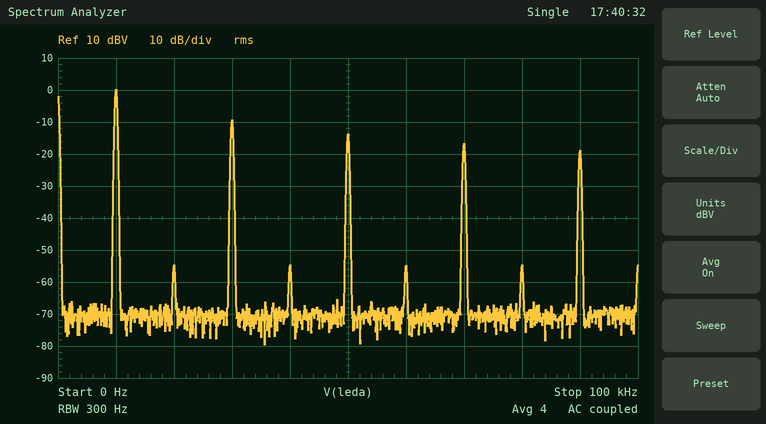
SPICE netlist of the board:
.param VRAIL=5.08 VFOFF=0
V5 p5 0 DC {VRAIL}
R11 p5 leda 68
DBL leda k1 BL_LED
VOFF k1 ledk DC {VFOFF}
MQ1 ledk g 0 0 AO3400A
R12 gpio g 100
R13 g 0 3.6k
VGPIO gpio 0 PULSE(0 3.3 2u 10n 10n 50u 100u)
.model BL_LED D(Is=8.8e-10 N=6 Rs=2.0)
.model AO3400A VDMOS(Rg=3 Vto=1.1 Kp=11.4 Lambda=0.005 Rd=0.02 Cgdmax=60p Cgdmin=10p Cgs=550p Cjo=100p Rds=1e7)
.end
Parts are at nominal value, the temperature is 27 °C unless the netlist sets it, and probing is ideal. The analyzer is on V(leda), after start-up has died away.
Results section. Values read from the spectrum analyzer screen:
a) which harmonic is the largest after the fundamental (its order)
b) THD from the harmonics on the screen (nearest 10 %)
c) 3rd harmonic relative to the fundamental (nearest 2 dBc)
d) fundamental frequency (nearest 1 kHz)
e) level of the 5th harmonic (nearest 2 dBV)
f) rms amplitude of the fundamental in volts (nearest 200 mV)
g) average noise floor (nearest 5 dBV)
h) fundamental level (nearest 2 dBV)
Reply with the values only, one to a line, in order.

3
40 %
-10 dBc
10 kHz
-14 dBV
1.0 V
-70 dBV
0 dBV
